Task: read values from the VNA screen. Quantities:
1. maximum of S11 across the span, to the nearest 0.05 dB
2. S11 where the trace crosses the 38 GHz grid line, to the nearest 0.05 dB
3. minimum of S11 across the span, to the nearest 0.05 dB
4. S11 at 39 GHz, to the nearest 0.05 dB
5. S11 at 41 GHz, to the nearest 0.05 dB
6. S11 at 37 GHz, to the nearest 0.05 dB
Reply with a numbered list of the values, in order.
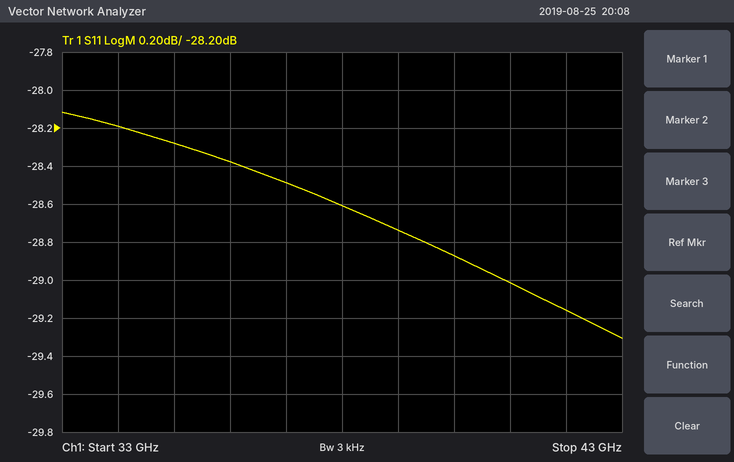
1. -28.10 dB
2. -28.60 dB
3. -29.30 dB
4. -28.75 dB
5. -29.00 dB
6. -28.50 dB
